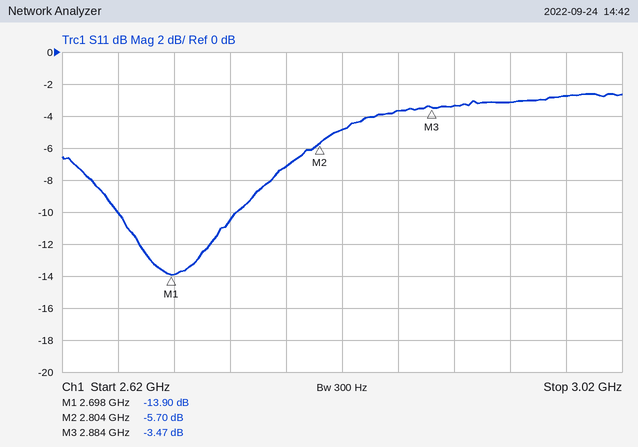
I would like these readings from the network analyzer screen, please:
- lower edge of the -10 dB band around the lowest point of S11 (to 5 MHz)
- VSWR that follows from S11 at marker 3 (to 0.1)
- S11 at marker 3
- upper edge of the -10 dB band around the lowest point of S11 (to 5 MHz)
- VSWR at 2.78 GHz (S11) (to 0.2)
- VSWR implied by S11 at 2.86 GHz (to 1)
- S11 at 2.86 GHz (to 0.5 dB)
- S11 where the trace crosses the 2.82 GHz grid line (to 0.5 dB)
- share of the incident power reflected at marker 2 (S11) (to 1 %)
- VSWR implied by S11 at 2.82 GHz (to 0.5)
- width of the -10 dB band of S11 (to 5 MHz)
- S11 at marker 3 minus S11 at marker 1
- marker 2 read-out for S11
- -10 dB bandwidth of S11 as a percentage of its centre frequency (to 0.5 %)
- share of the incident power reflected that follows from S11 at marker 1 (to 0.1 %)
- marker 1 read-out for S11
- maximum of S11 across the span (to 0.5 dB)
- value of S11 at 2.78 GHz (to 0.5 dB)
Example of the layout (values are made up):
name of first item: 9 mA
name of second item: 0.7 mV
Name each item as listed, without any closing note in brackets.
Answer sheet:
lower edge of the -10 dB band around the lowest point of S11: 2.660 GHz
VSWR that follows from S11 at marker 3: 5.1
S11 at marker 3: -3.47 dB
upper edge of the -10 dB band around the lowest point of S11: 2.745 GHz
VSWR at 2.78 GHz (S11): 2.6
VSWR implied by S11 at 2.86 GHz: 5
S11 at 2.86 GHz: -3.5 dB
S11 where the trace crosses the 2.82 GHz grid line: -5.0 dB
share of the incident power reflected at marker 2 (S11): 27 %
VSWR implied by S11 at 2.82 GHz: 3.5
width of the -10 dB band of S11: 85 MHz
S11 at marker 3 minus S11 at marker 1: 10.43 dB
marker 2 read-out for S11: -5.70 dB
-10 dB bandwidth of S11 as a percentage of its centre frequency: 3.0 %
share of the incident power reflected that follows from S11 at marker 1: 4.1 %
marker 1 read-out for S11: -13.90 dB
maximum of S11 across the span: -2.5 dB
value of S11 at 2.78 GHz: -7.0 dB
